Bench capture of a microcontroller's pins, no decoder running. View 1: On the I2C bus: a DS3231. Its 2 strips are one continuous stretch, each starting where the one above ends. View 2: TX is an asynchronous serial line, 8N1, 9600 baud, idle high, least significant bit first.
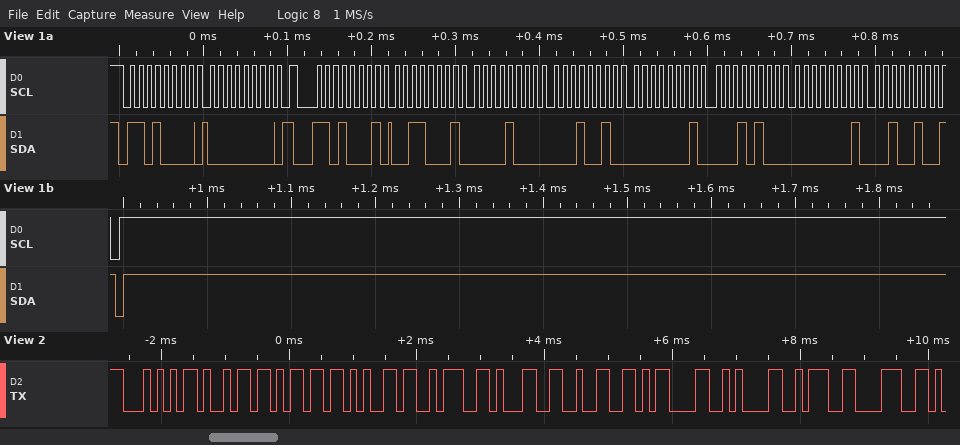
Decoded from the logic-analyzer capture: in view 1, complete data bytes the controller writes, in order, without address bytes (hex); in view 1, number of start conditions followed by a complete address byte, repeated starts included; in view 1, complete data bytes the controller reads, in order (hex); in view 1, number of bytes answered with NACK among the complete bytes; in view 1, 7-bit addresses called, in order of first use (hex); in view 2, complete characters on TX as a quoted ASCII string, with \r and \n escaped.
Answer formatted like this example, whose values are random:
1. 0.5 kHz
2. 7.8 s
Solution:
1. 00
2. 2
3. 31 08 12 01 14 01 24
4. 1
5. 0x68
6. "Time:12\r\n:8"
